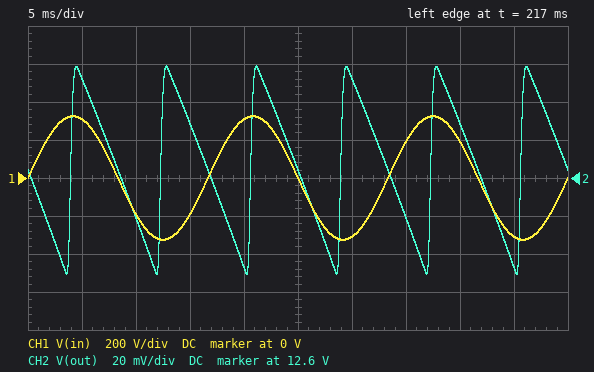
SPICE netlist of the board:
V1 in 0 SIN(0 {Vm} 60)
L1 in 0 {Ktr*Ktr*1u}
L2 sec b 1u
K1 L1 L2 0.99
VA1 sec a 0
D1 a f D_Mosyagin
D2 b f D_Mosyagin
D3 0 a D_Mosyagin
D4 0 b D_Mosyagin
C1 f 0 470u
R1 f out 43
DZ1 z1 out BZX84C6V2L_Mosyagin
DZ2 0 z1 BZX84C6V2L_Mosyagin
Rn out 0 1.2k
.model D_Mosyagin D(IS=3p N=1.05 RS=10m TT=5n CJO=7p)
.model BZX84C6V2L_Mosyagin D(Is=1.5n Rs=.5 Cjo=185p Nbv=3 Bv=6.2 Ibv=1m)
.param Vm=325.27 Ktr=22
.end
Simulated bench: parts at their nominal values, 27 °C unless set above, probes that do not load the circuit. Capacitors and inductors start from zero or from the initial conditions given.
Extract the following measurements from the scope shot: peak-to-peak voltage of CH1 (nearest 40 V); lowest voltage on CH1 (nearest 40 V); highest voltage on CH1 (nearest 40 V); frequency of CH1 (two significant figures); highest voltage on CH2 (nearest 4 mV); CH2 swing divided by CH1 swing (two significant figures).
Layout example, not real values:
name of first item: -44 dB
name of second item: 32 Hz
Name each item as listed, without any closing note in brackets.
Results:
peak-to-peak voltage of CH1: 640 V
lowest voltage on CH1: -320 V
highest voltage on CH1: 320 V
frequency of CH1: 60 Hz
highest voltage on CH2: 12.660 V
CH2 swing divided by CH1 swing: 0.00017
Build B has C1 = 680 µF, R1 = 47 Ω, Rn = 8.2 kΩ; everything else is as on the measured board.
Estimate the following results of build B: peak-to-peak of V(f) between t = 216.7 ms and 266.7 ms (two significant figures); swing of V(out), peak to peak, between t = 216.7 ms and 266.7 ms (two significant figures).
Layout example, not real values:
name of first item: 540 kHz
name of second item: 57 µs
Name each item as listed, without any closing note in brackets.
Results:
peak-to-peak of V(f) between t = 216.7 ms and 266.7 ms: 120 mV
swing of V(out), peak to peak, between t = 216.7 ms and 266.7 ms: 32 mV
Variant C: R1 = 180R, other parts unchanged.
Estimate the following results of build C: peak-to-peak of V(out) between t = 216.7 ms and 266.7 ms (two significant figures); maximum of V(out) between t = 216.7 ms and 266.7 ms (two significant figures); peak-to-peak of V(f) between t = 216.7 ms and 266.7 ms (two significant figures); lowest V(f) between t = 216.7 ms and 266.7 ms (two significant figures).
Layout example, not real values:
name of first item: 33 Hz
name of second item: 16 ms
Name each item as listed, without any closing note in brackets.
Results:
peak-to-peak of V(out) between t = 216.7 ms and 266.7 ms: 130 mV
maximum of V(out) between t = 216.7 ms and 266.7 ms: 12 V
peak-to-peak of V(f) between t = 216.7 ms and 266.7 ms: 150 mV
lowest V(f) between t = 216.7 ms and 266.7 ms: 13 V
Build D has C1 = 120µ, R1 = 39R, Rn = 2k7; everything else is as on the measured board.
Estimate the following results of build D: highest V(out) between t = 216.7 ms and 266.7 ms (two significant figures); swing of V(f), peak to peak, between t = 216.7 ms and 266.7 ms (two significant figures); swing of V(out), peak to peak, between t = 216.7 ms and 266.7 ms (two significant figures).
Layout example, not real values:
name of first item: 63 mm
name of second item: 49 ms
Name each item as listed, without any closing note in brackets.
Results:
highest V(out) between t = 216.7 ms and 266.7 ms: 13 V
swing of V(f), peak to peak, between t = 216.7 ms and 266.7 ms: 600 mV
swing of V(out), peak to peak, between t = 216.7 ms and 266.7 ms: 260 mV
